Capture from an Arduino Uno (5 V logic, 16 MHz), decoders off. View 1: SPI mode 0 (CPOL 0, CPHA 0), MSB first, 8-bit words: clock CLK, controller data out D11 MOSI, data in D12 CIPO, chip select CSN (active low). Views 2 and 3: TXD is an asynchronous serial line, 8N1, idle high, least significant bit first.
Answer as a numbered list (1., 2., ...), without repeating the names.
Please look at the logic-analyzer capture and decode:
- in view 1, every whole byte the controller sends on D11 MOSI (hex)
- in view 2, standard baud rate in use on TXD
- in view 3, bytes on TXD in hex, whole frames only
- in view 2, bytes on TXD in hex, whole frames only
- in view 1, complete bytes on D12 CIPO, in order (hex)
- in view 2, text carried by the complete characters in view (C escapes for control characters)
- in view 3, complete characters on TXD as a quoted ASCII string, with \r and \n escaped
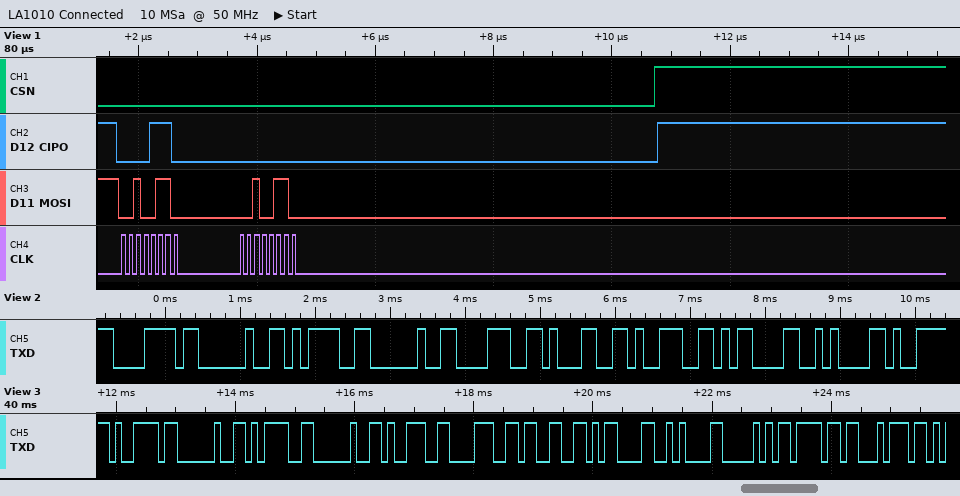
1. 26 26
2. 9600 baud
3. 0x79 0x20 0x3D 0x20 0x39 0x38 0x33 0x0D 0x0A 0x50 0x6F 0x74
4. 78 20 3D 20 38 31 39 0D 0A
5. 0E 00
6. "x = 819\r\n"
7. "y = 983\r\nPot"
